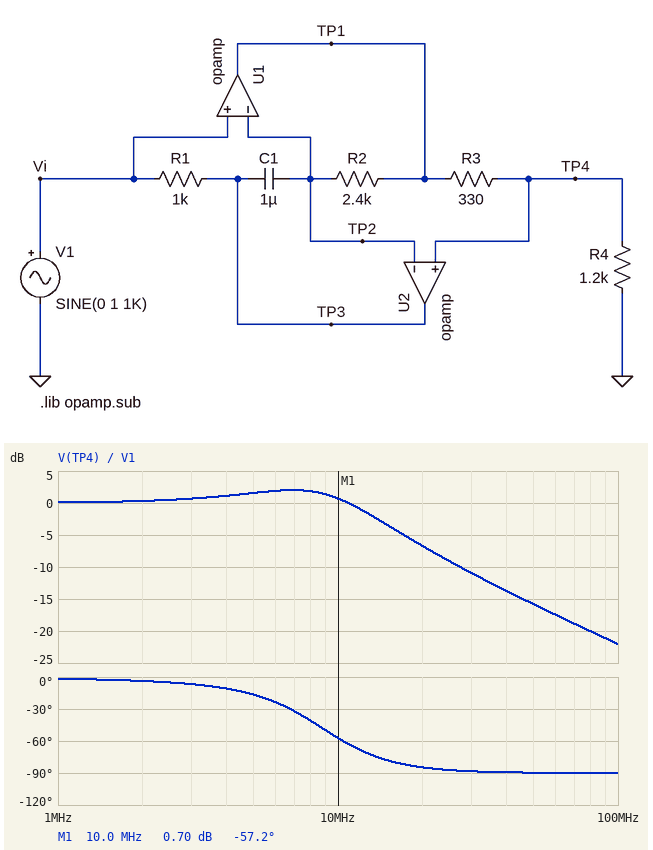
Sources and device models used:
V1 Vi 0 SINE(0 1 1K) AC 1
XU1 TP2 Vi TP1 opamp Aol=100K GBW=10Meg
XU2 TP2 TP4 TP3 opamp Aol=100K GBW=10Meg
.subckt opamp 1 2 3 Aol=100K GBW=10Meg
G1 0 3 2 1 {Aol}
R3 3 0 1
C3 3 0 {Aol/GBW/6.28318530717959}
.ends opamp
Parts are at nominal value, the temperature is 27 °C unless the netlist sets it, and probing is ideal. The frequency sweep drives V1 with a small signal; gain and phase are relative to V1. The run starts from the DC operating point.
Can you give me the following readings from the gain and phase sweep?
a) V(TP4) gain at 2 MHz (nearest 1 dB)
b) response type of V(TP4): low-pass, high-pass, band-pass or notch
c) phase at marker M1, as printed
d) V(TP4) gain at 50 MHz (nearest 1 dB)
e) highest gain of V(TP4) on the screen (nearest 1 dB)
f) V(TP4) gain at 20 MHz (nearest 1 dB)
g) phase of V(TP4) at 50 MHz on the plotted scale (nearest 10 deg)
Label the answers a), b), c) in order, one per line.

a) 0 dB
b) low-pass
c) -57.2 deg
d) -16 dB
e) 2 dB
f) -7 dB
g) -90 deg
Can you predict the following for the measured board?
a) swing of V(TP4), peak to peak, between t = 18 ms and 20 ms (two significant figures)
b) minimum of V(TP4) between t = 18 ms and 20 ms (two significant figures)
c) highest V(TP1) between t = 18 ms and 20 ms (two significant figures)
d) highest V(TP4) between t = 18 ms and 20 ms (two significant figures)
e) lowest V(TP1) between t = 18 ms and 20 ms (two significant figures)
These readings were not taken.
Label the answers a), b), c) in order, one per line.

a) 2.0 V
b) -1.0 V
c) 1.3 V
d) 1.0 V
e) -1.3 V
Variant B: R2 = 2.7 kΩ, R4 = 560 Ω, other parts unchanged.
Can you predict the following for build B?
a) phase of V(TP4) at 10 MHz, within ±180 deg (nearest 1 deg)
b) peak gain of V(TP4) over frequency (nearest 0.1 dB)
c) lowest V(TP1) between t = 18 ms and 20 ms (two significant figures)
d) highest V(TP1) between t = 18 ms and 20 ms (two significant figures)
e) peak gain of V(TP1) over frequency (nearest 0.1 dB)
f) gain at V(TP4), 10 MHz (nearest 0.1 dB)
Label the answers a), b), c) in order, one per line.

a) -65 deg
b) 1.0 dB
c) -1.6 V
d) 1.6 V
e) 5.0 dB
f) -1.6 dB
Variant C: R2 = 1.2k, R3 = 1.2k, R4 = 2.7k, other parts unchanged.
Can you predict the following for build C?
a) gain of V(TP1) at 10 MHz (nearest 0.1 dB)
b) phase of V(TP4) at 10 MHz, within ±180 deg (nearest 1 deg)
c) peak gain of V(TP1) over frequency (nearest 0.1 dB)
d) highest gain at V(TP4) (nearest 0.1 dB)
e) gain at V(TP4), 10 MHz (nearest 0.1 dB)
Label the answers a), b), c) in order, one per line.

a) 2.6 dB
b) -62 deg
c) 4.6 dB
d) 1.4 dB
e) -0.6 dB
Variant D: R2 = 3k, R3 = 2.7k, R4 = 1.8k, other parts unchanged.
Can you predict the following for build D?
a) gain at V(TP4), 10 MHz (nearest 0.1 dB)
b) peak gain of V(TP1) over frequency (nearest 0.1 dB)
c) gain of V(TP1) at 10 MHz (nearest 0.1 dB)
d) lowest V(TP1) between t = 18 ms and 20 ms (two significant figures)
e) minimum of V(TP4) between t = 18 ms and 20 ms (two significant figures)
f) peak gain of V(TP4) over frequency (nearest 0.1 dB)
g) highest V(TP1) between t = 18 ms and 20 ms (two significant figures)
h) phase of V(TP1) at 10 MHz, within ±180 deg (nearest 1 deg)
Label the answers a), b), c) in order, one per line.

a) -6.3 dB
b) 8.0 dB
c) 1.7 dB
d) -2.5 V
e) -1.0 V
f) 0 dB
g) 2.5 V
h) -76 deg
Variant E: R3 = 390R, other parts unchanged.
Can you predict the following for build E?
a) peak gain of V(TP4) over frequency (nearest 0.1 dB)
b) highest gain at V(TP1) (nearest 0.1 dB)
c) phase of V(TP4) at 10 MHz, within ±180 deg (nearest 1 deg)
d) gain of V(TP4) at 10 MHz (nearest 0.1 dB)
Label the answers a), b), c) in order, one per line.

a) 1.8 dB
b) 4.3 dB
c) -59 deg
d) 0.3 dB
